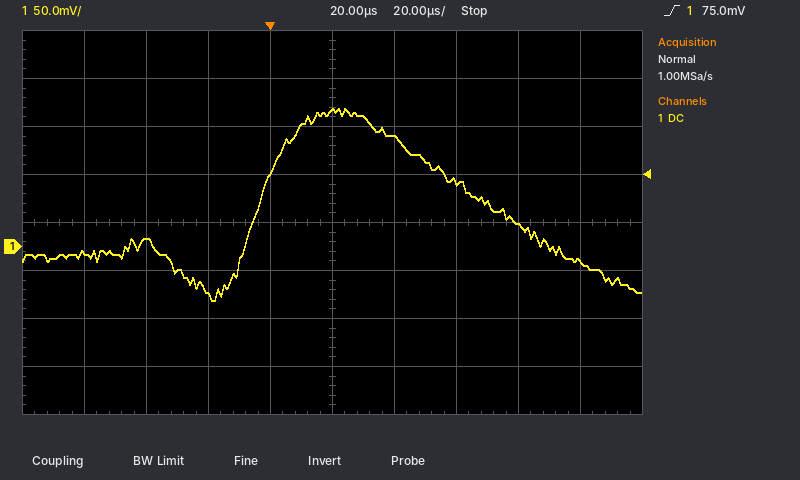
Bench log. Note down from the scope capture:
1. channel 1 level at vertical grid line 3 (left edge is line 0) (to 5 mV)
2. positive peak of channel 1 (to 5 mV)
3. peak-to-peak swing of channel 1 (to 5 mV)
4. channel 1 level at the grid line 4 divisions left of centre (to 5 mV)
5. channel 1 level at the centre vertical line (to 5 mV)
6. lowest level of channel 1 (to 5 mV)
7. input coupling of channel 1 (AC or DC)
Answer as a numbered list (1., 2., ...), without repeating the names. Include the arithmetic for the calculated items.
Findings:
1. -50 mV
2. 145 mV
3. 145 mV − (-55 mV) = 200 mV
4. -5 mV
5. 140 mV
6. -55 mV
7. DC
